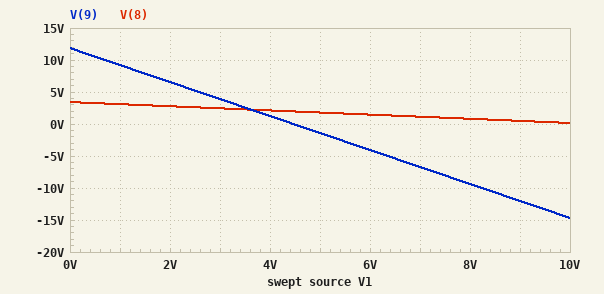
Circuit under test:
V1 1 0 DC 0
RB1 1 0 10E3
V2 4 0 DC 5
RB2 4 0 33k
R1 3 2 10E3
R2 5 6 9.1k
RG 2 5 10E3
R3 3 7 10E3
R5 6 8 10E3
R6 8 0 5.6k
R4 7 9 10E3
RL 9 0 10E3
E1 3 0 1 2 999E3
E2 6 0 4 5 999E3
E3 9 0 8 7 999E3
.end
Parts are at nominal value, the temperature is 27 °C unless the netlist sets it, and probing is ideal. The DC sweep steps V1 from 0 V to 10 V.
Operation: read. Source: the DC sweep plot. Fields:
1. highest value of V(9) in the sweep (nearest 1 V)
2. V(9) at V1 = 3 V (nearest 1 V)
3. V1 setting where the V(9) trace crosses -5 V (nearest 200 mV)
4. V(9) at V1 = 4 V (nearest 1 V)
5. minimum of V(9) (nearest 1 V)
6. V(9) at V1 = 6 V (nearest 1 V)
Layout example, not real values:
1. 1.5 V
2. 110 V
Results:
1. 12 V
2. 4 V
3. 6.4 V
4. 1 V
5. -15 V
6. -4 V
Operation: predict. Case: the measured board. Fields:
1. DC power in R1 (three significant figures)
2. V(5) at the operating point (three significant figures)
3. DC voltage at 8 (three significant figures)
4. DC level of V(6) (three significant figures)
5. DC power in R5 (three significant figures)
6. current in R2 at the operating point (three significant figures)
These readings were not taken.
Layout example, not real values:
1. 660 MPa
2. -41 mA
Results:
1. 2.50 mW
2. 5.00 V
3. 3.43 V
4. 9.55 V
5. 3.75 mW
6. 500 µA
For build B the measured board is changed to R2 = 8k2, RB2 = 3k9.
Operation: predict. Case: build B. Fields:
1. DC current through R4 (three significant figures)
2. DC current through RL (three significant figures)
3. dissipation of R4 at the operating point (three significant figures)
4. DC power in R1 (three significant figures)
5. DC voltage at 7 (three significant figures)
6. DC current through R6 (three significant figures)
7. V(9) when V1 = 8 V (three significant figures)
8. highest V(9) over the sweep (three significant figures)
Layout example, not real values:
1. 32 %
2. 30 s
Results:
1. 827 µA
2. 1.15 mA
3. 6.83 mW
4. 2.50 mW
5. 3.27 V
6. 583 µA
7. -9.18 V
8. 11.5 V
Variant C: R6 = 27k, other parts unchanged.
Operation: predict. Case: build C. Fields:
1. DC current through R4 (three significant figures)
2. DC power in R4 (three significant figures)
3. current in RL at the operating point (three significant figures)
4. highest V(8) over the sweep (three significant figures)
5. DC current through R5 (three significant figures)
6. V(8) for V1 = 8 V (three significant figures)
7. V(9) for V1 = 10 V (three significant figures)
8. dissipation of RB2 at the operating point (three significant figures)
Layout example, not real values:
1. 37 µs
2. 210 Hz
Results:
1. 1.20 mA
2. 14.3 mW
3. 1.89 mA
4. 6.97 V
5. 258 µA
6. 1.66 V
7. -14.3 V
8. 758 µW
